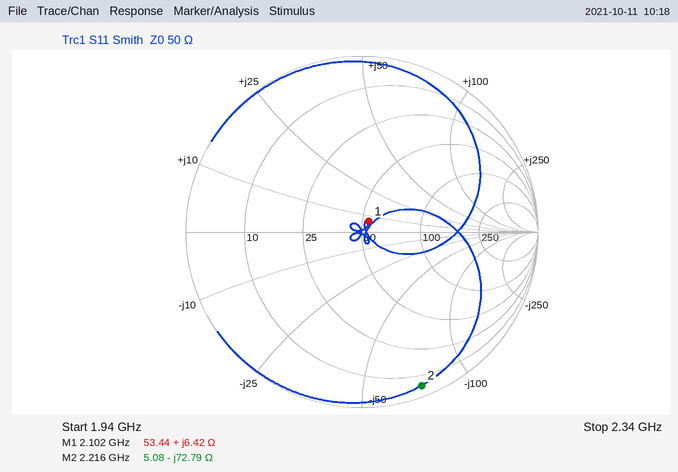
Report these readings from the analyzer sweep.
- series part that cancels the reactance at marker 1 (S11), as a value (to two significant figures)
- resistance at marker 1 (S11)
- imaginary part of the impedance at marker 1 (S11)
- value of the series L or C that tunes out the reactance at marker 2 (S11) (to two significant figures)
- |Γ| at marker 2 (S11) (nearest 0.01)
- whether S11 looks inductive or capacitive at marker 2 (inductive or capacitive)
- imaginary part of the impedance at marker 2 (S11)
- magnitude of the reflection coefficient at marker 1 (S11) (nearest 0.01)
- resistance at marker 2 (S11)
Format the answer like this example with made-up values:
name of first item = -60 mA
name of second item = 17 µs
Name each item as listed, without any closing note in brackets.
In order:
series part that cancels the reactance at marker 1 (S11), as a value = 12 pF
resistance at marker 1 = 53.44 Ω
imaginary part of the impedance at marker 1 = +6.42 Ω
value of the series L or C that tunes out the reactance at marker 2 (S11) = 5.2 nH
|Γ| at marker 2 (S11) = 0.94
whether S11 looks inductive or capacitive at marker 2 = capacitive
imaginary part of the impedance at marker 2 = -72.79 Ω
magnitude of the reflection coefficient at marker 1 (S11) = 0.07
resistance at marker 2 = 5.08 Ω
